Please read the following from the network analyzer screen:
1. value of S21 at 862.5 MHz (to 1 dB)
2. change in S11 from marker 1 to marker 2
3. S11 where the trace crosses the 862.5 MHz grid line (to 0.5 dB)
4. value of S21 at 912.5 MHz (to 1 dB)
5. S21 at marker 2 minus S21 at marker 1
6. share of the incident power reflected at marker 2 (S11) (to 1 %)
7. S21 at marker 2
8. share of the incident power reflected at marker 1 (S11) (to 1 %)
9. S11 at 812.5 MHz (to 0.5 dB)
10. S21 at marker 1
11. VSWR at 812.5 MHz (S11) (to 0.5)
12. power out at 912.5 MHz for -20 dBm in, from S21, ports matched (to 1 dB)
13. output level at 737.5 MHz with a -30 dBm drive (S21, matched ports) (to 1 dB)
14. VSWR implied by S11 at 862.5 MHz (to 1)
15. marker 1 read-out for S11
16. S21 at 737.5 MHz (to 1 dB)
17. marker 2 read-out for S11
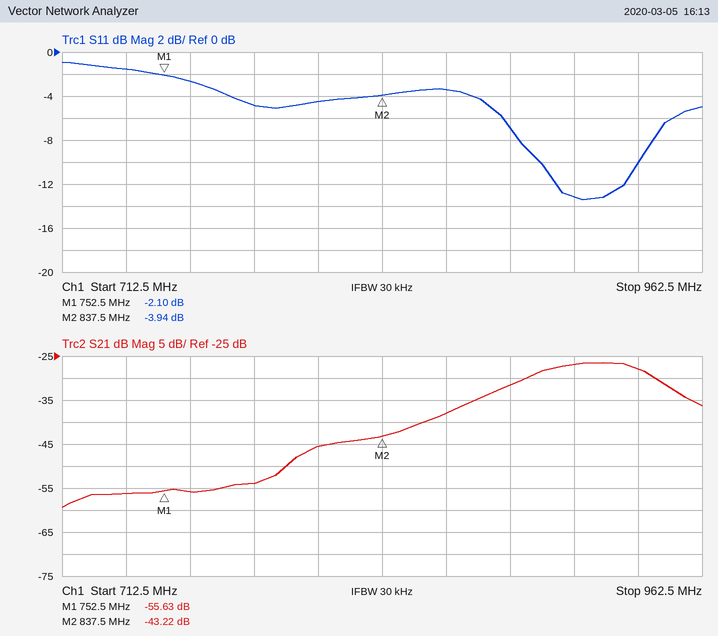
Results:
-38 dB
-1.84 dB
-3.5 dB
-27 dB
12.41 dB
40 %
-43.22 dB
62 %
-4.5 dB
-55.63 dB
4.0
-47 dBm
-86 dBm
5
-2.10 dB
-56 dB
-3.94 dB
